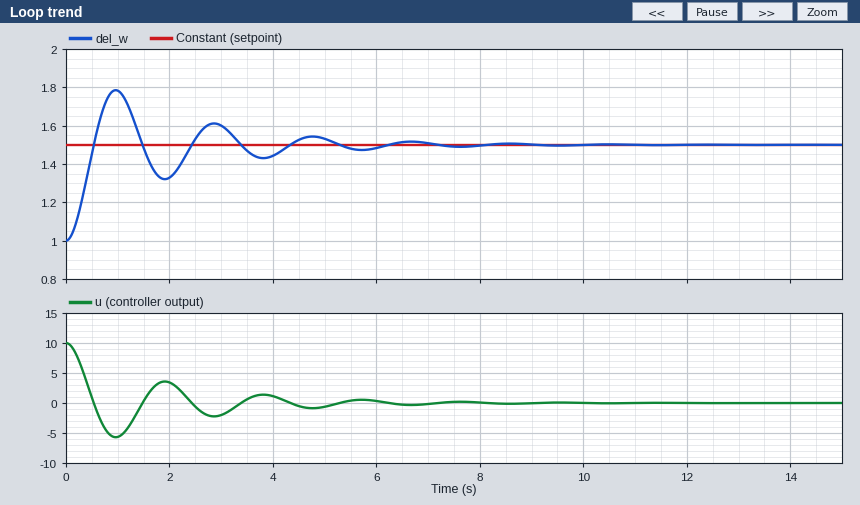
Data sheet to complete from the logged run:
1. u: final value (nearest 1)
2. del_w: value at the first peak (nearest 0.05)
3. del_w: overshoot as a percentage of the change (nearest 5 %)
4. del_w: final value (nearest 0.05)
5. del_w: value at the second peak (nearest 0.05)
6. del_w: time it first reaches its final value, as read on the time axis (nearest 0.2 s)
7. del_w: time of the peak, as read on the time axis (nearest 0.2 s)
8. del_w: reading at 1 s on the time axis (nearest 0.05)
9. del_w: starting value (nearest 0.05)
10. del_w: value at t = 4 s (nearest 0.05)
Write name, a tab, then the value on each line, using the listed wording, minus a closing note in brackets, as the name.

u: final value	0
del_w: value at the first peak	1.80
del_w: overshoot as a percentage of the change	55 %
del_w: final value	1.50
del_w: value at the second peak	1.60
del_w: time it first reaches its final value, as read on the time axis	0.6 s
del_w: time of the peak, as read on the time axis	1.0 s
del_w: reading at 1 s on the time axis	1.80
del_w: starting value	1.00
del_w: value at t = 4 s	1.45
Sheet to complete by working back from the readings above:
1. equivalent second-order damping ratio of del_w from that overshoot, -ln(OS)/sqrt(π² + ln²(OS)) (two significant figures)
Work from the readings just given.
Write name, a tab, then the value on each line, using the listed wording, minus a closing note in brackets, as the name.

equivalent second-order damping ratio of del_w from that overshoot, -ln(OS)/sqrt(π² + ln²(OS))	0.19
